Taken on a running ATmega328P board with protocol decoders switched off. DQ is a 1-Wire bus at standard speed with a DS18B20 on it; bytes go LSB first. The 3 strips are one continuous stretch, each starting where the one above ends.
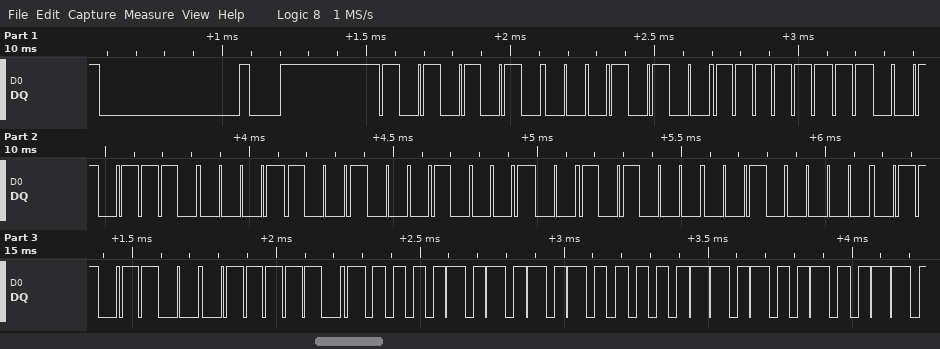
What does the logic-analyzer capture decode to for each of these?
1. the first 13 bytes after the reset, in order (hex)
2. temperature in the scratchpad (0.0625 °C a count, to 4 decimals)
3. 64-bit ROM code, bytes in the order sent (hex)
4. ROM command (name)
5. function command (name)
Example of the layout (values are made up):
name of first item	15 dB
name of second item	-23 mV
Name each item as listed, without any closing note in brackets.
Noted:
the first 13 bytes after the reset, in order	55 28 FF 74 98 88 14 04 36 BE 50 05 4B
temperature in the scratchpad	85.0000 °C
64-bit ROM code, bytes in the order sent	28 FF 74 98 88 14 04 36
ROM command	Match ROM
function command	Read Scratchpad
